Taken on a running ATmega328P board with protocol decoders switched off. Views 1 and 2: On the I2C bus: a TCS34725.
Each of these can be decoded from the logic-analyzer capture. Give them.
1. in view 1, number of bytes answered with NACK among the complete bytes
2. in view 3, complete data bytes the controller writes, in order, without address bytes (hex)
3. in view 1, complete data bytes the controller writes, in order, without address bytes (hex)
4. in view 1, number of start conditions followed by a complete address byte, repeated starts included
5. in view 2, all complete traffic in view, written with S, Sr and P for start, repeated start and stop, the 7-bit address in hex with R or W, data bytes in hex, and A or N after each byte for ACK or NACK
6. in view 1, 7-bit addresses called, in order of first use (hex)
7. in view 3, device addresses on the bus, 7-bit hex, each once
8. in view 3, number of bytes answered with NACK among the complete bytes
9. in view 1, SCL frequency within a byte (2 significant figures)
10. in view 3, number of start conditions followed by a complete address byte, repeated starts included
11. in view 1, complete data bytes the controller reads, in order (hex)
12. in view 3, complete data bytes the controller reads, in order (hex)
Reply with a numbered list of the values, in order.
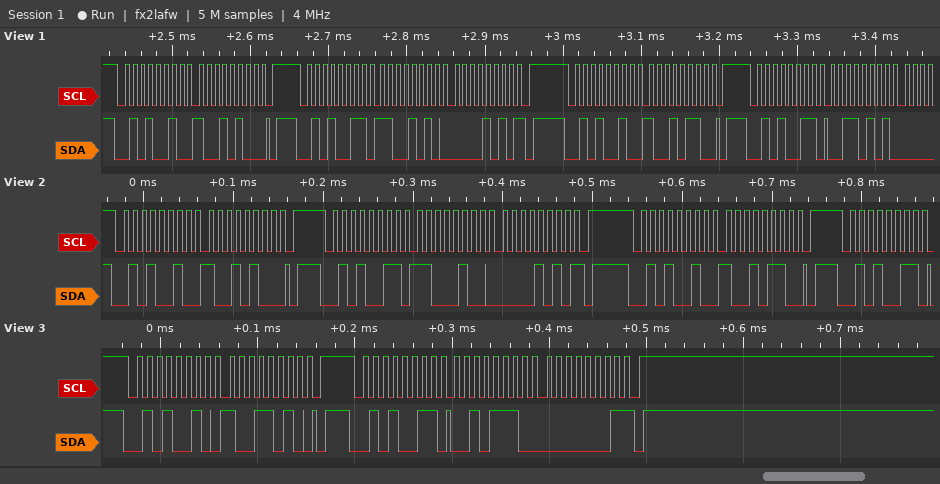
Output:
1. 1
2. 9A
3. 94 96
4. 4
5. S 29W A 94 A P S 29R A C4 A 0A N P S 29W A 96 A P S 29R A
6. 0x29
7. 0x29
8. 1
9. 100 kHz
10. 2
11. CA 0A 35
12. 2E 01
